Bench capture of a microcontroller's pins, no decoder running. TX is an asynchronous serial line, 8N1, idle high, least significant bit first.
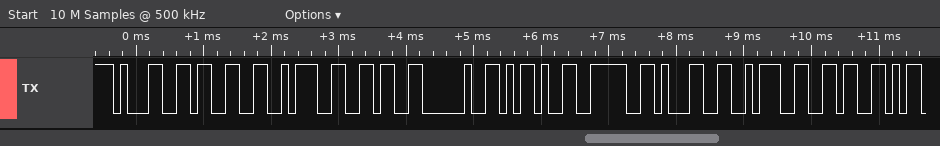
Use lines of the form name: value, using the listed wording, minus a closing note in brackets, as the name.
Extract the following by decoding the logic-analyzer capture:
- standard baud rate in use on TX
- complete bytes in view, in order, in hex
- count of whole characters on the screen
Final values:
standard baud rate in use on TX: 9600 baud
complete bytes in view, in order, in hex: 0x31 0x33 0x3A 0x36 0x20 0x2D 0x3E 0x31 0x3A 0x36
count of whole characters on the screen: 10
